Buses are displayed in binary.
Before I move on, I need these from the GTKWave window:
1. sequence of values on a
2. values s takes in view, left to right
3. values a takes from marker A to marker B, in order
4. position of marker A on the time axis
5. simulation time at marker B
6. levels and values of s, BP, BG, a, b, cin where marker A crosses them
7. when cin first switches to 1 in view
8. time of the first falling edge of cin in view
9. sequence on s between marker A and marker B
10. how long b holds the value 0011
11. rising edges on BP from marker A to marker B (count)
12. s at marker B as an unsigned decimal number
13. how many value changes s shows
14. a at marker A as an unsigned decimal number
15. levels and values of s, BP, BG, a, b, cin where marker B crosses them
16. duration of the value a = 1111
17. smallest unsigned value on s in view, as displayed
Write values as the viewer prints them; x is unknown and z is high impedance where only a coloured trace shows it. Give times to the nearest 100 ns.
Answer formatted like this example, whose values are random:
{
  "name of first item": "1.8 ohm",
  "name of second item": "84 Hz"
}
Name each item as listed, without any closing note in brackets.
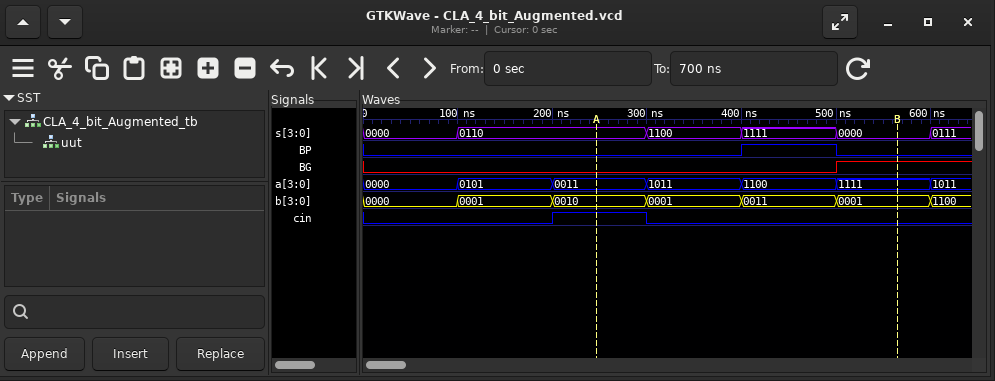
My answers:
{
  "sequence of values on a": "0000, 0101, 0011, 1011, 1100, 1111, 1011",
  "values s takes in view, left to right": "0000, 0110, 1100, 1111, 0000, 0111",
  "values a takes from marker A to marker B, in order": "0011, 1011, 1100, 1111",
  "position of marker A on the time axis": "200 ns",
  "simulation time at marker B": "600 ns",
  "levels and values of s, BP, BG, a, b, cin where marker A crosses them": "s=0110, BP=0, BG=0, a=0011, b=0010, cin=1",
  "when cin first switches to 1 in view": "200 ns",
  "time of the first falling edge of cin in view": "300 ns",
  "sequence on s between marker A and marker B": "0110, 1100, 1111, 0000",
  "how long b holds the value 0011": "100 ns",
  "rising edges on BP from marker A to marker B": "1",
  "s at marker B as an unsigned decimal number": "0",
  "how many value changes s shows": "5",
  "a at marker A as an unsigned decimal number": "3",
  "levels and values of s, BP, BG, a, b, cin where marker B crosses them": "s=0000, BP=0, BG=1, a=1111, b=0001, cin=0",
  "duration of the value a = 1111": "100 ns",
  "smallest unsigned value on s in view, as displayed": "0000"
}
